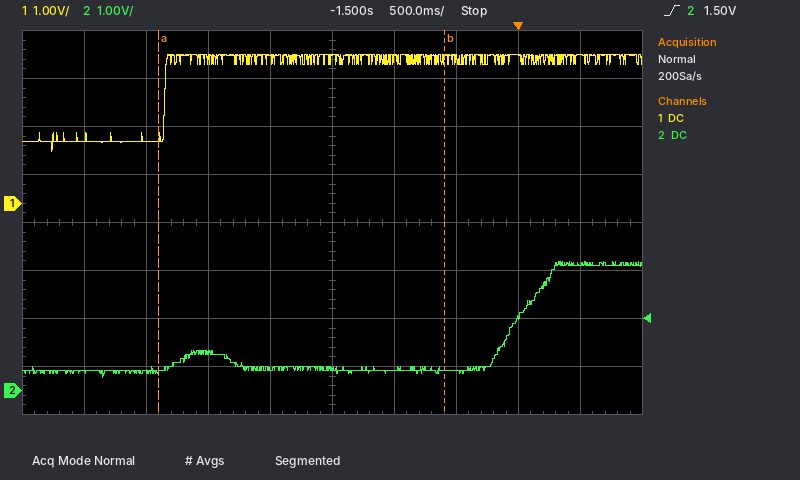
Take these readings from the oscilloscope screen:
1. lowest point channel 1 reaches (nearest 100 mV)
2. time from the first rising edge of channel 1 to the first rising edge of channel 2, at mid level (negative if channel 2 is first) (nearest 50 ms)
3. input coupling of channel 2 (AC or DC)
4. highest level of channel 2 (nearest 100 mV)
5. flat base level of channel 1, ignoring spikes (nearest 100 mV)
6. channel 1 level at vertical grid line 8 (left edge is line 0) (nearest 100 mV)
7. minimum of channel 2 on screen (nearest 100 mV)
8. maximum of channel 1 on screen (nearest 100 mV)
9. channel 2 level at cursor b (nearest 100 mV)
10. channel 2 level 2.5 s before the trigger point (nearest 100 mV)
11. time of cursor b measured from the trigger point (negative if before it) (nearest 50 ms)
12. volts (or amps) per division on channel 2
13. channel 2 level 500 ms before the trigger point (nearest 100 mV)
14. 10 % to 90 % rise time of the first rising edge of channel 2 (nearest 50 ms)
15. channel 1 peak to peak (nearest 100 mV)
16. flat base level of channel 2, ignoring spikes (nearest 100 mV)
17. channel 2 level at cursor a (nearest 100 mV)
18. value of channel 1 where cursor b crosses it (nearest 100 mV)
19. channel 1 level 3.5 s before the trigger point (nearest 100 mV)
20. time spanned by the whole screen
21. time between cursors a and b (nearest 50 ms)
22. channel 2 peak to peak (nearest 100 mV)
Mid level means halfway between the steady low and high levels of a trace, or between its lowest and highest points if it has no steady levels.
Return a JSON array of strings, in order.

["1.1 V", "+2.85 s", "DC", "2.7 V", "1.3 V", "3.0 V", "300 mV", "3.1 V", "400 mV", "800 mV", "-600 ms", "1 V", "400 mV", "450 ms", "2.0 V", "400 mV", "400 mV", "3.0 V", "1.4 V", "5 s", "2.30 s", "2.4 V"]
